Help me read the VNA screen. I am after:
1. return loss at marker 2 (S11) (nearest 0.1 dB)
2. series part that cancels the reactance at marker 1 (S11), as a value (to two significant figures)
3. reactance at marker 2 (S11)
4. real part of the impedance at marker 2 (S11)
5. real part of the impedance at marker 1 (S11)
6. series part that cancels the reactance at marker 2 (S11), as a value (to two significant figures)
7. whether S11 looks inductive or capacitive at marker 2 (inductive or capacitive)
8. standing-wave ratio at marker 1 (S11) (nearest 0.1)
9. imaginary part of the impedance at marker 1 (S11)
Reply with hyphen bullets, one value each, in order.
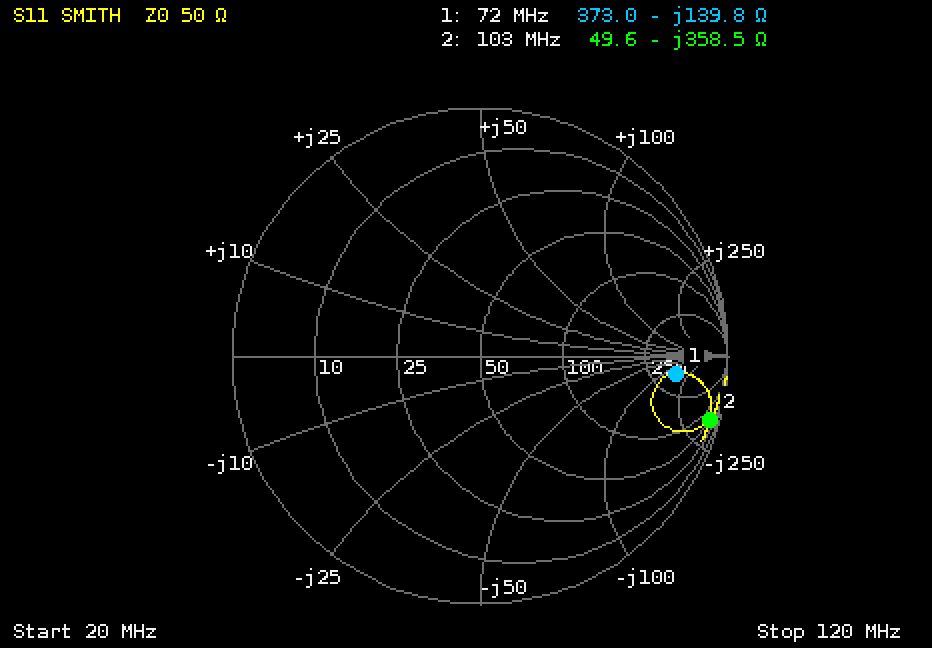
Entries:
- 0.3 dB
- 310 nH
- -358.5 Ω
- 49.6 Ω
- 373.0 Ω
- 550 nH
- capacitive
- 8.5
- -139.8 Ω
